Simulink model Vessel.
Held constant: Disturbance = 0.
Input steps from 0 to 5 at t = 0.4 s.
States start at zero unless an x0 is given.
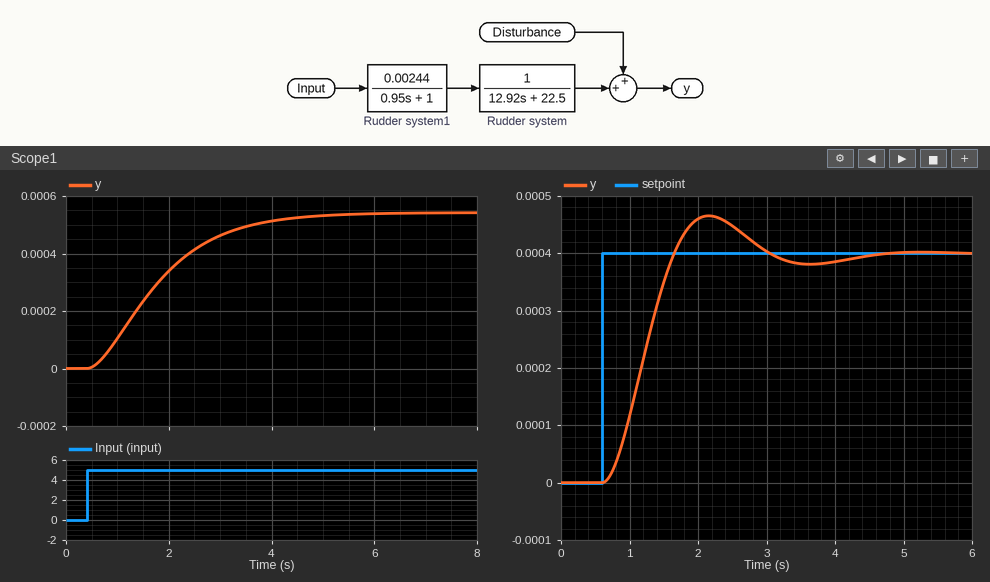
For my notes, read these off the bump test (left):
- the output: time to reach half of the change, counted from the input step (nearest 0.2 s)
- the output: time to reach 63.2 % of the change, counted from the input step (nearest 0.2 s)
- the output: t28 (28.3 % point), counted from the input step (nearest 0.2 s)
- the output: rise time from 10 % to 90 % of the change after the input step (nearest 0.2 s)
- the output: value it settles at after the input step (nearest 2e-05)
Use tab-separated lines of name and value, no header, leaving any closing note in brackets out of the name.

the output: time to reach half of the change, counted from the input step	1.2 s
the output: time to reach 63.2 % of the change, counted from the input step	1.6 s
the output: t28 (28.3 % point), counted from the input step	0.8 s
the output: rise time from 10 % to 90 % of the change after the input step	2.6 s
the output: value it settles at after the input step	0.00054
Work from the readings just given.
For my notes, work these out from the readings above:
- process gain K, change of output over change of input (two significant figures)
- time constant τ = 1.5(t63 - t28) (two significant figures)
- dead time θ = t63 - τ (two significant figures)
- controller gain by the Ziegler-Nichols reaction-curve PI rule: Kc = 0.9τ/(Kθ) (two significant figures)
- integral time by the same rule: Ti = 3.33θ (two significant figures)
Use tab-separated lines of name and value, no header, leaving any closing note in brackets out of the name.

process gain K, change of output over change of input	0.00011
time constant τ = 1.5(t63 - t28)	1.2 s
dead time θ = t63 - τ	0.40 s
controller gain by the Ziegler-Nichols reaction-curve PI rule: Kc = 0.9τ/(Kθ)	25000
integral time by the same rule: Ti = 3.33θ	1.3 s
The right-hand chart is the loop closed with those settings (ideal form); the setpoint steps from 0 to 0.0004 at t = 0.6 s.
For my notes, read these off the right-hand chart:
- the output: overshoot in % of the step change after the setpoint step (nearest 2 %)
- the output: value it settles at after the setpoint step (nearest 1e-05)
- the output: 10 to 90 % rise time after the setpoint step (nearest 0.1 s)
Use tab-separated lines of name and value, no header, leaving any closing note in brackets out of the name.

the output: overshoot in % of the step change after the setpoint step	16 %
the output: value it settles at after the setpoint step	0.00040
the output: 10 to 90 % rise time after the setpoint step	0.7 s
